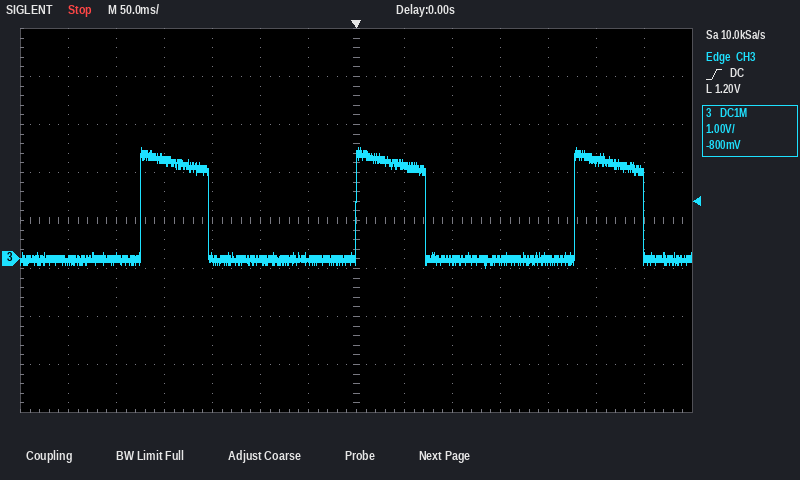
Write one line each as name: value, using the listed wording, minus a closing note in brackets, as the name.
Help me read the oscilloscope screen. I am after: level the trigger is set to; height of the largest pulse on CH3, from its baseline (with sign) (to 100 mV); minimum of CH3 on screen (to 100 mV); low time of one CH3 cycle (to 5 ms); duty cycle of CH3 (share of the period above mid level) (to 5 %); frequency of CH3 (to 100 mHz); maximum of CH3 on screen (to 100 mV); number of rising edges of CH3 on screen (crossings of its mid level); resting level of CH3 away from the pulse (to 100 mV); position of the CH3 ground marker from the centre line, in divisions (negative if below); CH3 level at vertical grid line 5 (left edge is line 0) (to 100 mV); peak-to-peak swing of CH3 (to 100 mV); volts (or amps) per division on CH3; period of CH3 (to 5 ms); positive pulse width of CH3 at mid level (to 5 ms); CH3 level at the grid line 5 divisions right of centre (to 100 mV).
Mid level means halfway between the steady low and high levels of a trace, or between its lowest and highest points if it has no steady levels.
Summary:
level the trigger is set to: 1.20 V
height of the largest pulse on CH3, from its baseline (with sign): +2.3 V
minimum of CH3 on screen: -200 mV
low time of one CH3 cycle: 155 ms
duty cycle of CH3 (share of the period above mid level): 30 %
frequency of CH3: 4.4 Hz
maximum of CH3 on screen: 2.3 V
number of rising edges of CH3 on screen: 3
resting level of CH3 away from the pulse: 0.0 V
position of the CH3 ground marker from the centre line, in divisions: -0.8 div
CH3 level at vertical grid line 5 (left edge is line 0): 0.0 V
peak-to-peak swing of CH3: 2.5 V
volts (or amps) per division on CH3: 1 V
period of CH3: 225 ms
positive pulse width of CH3 at mid level: 70 ms
CH3 level at the grid line 5 divisions right of centre: 2.0 V
